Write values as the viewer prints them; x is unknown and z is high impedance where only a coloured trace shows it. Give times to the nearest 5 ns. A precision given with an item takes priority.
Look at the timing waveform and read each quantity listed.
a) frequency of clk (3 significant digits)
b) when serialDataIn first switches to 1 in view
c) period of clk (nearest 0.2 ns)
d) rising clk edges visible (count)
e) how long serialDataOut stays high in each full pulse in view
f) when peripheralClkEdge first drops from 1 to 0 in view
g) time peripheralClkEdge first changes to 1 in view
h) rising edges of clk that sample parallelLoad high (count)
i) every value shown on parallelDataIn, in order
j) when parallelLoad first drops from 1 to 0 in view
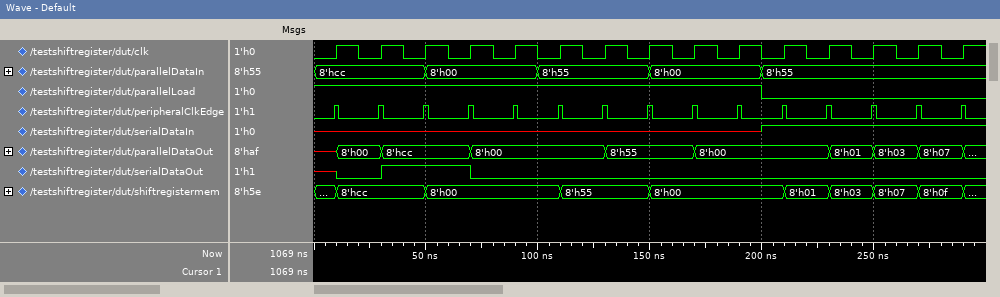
50.0 MHz
200 ns
20 ns
15
40 ns
10 ns
10 ns
10
8'hcc, 8'h00, 8'h55, 8'h00, 8'h55
200 ns
